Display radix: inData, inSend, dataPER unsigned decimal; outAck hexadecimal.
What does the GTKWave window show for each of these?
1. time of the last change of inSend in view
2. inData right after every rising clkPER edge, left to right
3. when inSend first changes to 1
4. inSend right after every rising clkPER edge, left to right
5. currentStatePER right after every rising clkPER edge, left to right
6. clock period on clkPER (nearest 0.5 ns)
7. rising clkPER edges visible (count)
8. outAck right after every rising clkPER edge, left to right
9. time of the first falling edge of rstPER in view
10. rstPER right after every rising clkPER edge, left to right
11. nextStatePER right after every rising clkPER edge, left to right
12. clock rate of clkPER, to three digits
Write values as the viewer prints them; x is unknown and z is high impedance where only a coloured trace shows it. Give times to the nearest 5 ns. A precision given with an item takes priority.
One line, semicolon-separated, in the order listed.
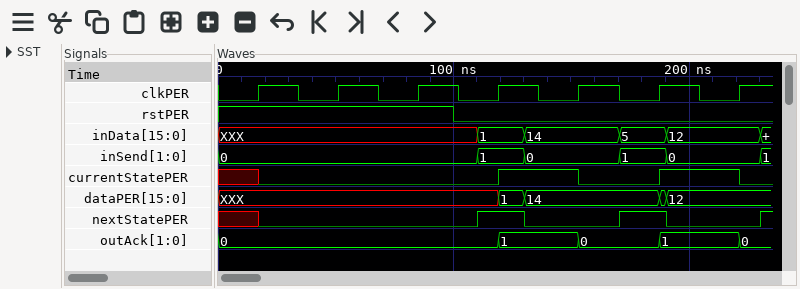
230 ns; XXX, XXX, XXX, 1, 14, 5, 12; 110 ns; 0, 0, 0, 1, 0, 1, 0; 0 0 0 1 0 1 0; 34 ns; 7; 0, 0, 0, 1, 0, 1, 0; 100 ns; 1 1 1 0 0 0 0; 0 0 0 1 0 1 0; 29.4 MHz
